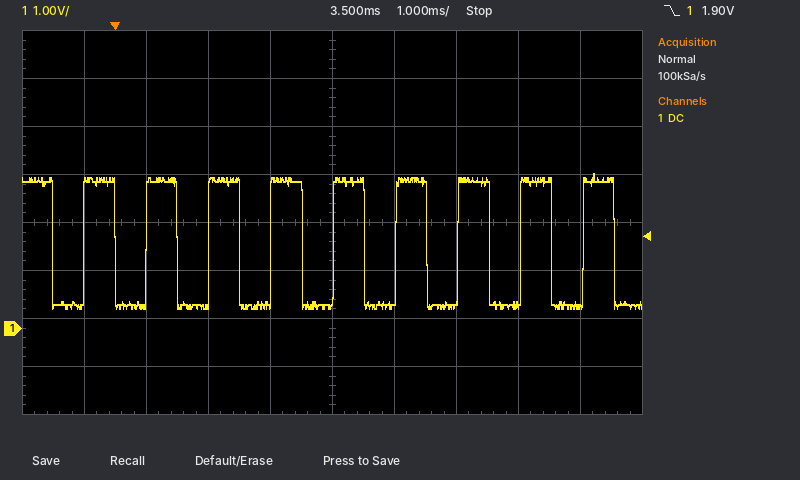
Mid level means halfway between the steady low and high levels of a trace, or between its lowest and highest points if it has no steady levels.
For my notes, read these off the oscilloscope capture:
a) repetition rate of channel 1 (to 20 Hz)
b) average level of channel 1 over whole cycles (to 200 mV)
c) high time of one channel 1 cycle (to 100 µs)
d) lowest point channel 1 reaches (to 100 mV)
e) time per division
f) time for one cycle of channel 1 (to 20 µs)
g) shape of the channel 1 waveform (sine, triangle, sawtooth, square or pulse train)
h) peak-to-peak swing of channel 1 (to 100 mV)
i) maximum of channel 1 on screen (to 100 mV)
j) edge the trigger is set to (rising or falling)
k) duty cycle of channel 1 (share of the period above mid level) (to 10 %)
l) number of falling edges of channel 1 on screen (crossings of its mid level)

1.00 kHz
1.8 V
500 µs
400 mV
1 ms
1.00 ms
square
2.8 V
3.2 V
falling
50 %
10
